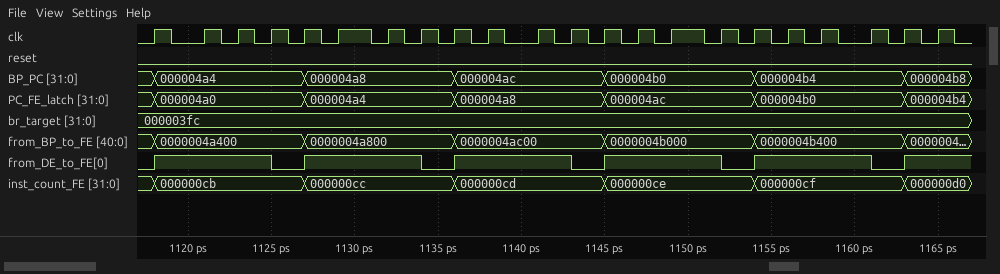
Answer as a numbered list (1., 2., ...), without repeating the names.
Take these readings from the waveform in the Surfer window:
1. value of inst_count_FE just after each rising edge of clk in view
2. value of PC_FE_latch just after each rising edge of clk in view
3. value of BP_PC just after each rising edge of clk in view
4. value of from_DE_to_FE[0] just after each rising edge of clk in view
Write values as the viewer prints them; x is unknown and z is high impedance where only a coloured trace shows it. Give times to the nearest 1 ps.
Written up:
1. 000000cb, 000000cb, 000000cb, 000000cb, 000000cc, 000000cc, 000000cc, 000000cc, 000000cd, 000000cd, 000000cd, 000000cd, 000000ce, 000000ce, 000000ce, 000000ce, 000000cf, 000000cf, 000000cf, 000000cf, 000000d0, 000000d0
2. 000004a0, 000004a0, 000004a0, 000004a0, 000004a4, 000004a4, 000004a4, 000004a4, 000004a8, 000004a8, 000004a8, 000004a8, 000004ac, 000004ac, 000004ac, 000004ac, 000004b0, 000004b0, 000004b0, 000004b0, 000004b4, 000004b4
3. 000004a4, 000004a4, 000004a4, 000004a4, 000004a8, 000004a8, 000004a8, 000004a8, 000004ac, 000004ac, 000004ac, 000004ac, 000004b0, 000004b0, 000004b0, 000004b0, 000004b4, 000004b4, 000004b4, 000004b4, 000004b8, 000004b8
4. 1 1 1 0 1 1 1 0 1 1 1 0 1 1 1 0 1 1 1 0 1 1
